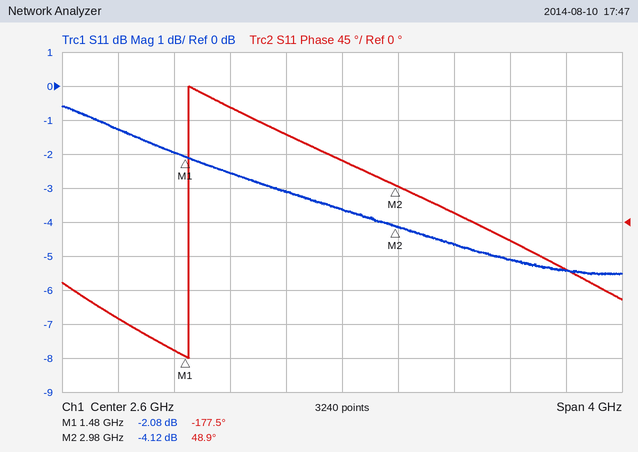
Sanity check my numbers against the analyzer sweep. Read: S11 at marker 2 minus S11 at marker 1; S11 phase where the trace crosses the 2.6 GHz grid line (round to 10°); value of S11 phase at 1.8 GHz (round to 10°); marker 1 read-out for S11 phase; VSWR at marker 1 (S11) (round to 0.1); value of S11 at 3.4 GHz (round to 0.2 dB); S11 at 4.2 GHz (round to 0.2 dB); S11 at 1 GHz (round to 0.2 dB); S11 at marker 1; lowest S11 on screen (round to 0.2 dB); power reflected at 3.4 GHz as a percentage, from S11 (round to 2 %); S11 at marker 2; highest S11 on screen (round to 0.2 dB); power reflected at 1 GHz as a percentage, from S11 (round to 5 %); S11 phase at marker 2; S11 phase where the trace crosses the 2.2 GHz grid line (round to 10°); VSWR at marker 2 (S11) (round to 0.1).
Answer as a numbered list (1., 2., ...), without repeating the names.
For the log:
1. -2.04 dB
2. 80°
3. 150°
4. -177.5°
5. 8.4
6. -4.6 dB
7. -5.4 dB
8. -1.2 dB
9. -2.08 dB
10. -5.6 dB
11. 34 %
12. -4.12 dB
13. -0.6 dB
14. 75 %
15. 48.9°
16. 120°
17. 4.3
